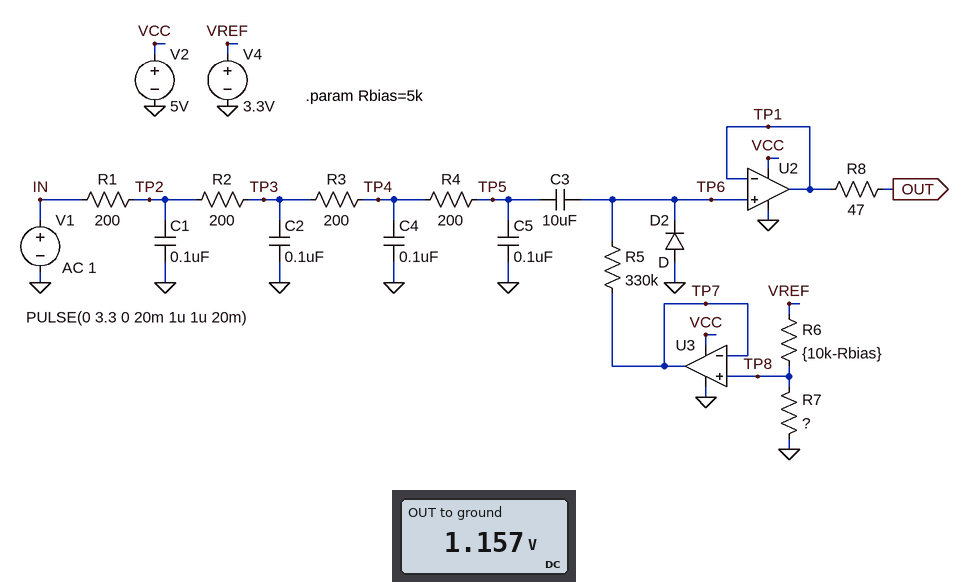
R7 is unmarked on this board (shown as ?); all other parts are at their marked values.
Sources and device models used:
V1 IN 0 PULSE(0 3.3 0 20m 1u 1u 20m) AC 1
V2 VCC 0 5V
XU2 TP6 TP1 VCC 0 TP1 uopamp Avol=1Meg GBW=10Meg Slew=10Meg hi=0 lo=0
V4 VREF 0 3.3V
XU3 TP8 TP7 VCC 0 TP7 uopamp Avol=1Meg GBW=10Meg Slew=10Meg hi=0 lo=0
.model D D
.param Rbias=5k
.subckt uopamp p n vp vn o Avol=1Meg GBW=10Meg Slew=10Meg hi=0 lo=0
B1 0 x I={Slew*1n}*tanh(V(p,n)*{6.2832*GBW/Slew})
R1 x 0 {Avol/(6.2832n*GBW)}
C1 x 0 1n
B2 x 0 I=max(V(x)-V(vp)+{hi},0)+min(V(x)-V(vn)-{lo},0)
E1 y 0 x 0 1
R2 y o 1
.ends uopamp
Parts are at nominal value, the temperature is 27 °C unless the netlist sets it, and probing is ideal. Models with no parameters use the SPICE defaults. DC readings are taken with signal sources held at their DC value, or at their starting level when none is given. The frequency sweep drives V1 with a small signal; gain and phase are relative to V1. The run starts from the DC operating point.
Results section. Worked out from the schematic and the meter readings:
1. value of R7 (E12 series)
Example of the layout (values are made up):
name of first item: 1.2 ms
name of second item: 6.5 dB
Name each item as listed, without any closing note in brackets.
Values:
value of R7: 2.7 kΩ
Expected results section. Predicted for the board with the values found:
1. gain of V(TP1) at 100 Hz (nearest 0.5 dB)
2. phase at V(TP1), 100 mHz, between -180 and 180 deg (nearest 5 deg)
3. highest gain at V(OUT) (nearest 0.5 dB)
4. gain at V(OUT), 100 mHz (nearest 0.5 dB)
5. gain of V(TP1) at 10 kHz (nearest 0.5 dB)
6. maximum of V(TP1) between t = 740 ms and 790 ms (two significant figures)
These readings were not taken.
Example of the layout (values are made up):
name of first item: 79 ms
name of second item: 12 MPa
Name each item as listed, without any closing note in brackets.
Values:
gain of V(TP1) at 100 Hz: 0 dB
phase at V(TP1), 100 mHz, between -180 and 180 deg: 25 deg
highest gain at V(OUT): 0 dB
gain at V(OUT), 100 mHz: -1.0 dB
gain of V(TP1) at 10 kHz: -26.0 dB
maximum of V(TP1) between t = 740 ms and 790 ms: 4.1 V
